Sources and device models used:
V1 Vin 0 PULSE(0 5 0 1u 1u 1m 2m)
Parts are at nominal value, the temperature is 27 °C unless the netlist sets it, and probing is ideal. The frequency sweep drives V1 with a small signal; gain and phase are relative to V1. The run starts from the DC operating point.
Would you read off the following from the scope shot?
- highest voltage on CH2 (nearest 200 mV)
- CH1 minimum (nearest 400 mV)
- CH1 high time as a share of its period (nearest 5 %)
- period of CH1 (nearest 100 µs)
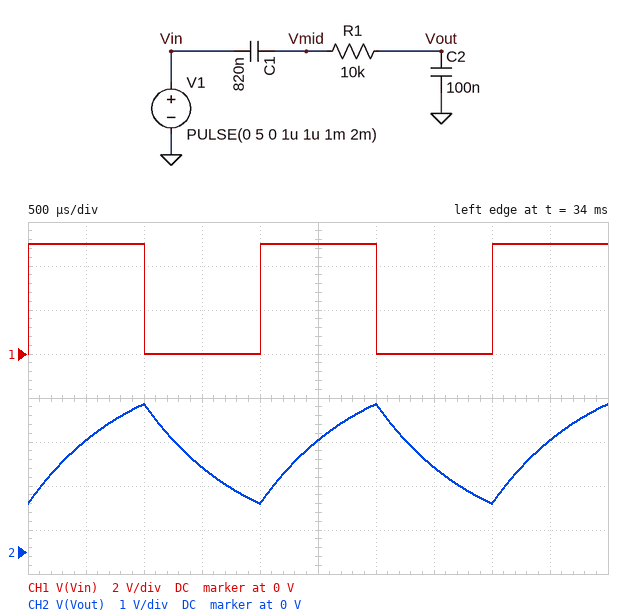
3.4 V
0 V
50 %
2.0 ms
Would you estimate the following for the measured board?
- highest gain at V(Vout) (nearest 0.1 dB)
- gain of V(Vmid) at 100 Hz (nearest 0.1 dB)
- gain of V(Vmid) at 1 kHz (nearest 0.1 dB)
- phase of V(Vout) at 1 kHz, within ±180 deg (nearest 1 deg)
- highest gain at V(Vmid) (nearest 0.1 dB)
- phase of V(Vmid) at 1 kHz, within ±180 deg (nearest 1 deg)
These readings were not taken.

-1.0 dB
-0.7 dB
0 dB
-80 deg
0 dB
1 deg
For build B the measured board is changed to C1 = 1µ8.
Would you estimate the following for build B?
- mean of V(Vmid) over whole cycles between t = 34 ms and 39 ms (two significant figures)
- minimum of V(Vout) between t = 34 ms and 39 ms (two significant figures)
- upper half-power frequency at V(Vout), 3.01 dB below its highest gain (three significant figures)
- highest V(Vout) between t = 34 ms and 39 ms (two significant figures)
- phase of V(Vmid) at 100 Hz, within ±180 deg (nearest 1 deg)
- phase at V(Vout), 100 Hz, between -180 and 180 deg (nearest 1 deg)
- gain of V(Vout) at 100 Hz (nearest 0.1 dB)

2.4 V
1.2 V
168 Hz
3.5 V
1 deg
-31 deg
-1.8 dB
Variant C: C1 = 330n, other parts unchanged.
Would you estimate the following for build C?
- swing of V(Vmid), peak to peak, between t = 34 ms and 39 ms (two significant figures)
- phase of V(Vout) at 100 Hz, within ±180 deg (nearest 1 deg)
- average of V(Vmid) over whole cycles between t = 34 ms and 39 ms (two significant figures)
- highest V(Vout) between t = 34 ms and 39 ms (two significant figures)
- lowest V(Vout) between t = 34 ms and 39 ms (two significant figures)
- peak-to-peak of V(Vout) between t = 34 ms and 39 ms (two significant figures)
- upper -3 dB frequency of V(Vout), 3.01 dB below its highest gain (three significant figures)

5.7 V
-26 deg
1.9 V
3.0 V
820 mV
2.2 V
207 Hz
